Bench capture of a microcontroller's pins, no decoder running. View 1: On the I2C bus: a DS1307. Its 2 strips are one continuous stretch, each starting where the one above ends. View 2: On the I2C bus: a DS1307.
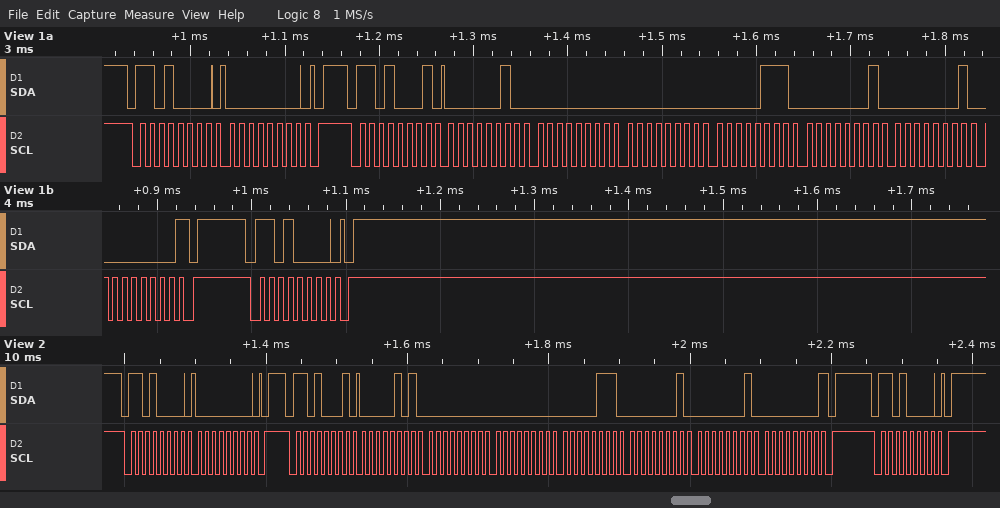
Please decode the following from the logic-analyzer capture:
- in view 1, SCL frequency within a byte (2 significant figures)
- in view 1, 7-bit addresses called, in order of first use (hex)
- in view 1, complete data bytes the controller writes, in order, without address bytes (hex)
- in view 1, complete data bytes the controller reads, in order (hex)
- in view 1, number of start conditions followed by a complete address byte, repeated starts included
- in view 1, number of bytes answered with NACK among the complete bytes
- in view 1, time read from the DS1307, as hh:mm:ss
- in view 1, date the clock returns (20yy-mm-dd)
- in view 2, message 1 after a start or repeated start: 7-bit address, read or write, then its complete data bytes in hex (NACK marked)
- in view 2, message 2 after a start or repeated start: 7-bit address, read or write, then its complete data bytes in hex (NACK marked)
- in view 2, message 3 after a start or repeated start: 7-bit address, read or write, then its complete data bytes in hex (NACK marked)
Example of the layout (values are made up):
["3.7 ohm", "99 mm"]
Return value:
["100 kHz", "0x68", "00", "02 00 00 07 01 01 00", "3", "1", "00:00:02", "2000-01-01", "0x68 write: 00", "0x68 read: 05 00 00 07 01 01 00 NACK", "0x68 write"]
